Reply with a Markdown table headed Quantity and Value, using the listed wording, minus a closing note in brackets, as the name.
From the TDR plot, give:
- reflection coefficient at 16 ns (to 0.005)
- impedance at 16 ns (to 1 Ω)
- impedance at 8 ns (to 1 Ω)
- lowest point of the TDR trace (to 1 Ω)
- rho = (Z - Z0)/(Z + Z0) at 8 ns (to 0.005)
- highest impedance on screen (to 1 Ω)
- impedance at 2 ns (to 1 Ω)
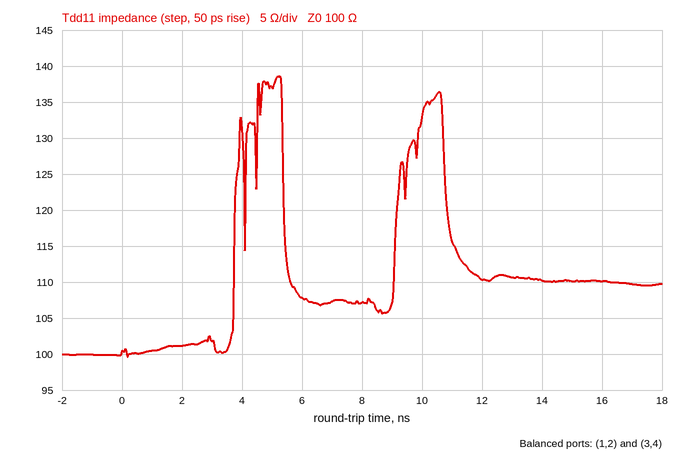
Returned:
| Quantity | Value |
|---|---|
| reflection coefficient at 16 ns | +0.050 |
| impedance at 16 ns | 110 Ω |
| impedance at 8 ns | 107 Ω |
| lowest point of the TDR trace | 100 Ω |
| rho = (Z - Z0)/(Z + Z0) at 8 ns | +0.035 |
| highest impedance on screen | 139 Ω |
| impedance at 2 ns | 101 Ω |
